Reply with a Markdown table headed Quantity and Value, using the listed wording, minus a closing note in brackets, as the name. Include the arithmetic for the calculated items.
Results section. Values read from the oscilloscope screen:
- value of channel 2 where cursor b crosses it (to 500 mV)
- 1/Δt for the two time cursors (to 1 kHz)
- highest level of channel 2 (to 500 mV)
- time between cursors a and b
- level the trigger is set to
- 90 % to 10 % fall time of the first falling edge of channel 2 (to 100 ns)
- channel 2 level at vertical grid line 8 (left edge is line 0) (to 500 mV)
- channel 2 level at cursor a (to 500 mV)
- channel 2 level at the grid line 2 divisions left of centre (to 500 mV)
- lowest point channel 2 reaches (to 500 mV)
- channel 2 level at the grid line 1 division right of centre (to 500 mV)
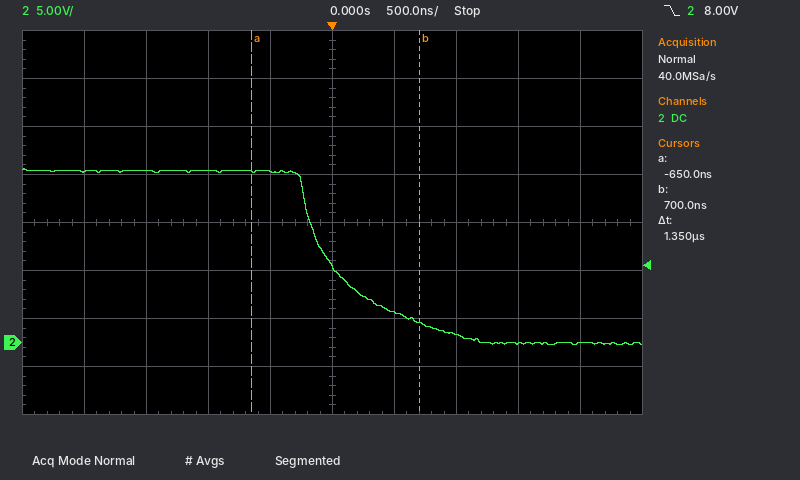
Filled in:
| Quantity | Value |
|---|---|
| value of channel 2 where cursor b crosses it | 2.0 V |
| 1/Δt for the two time cursors | 1 / 1.35 µs ≈ 741 kHz |
| highest level of channel 2 | 18.0 V |
| time between cursors a and b | 1.35 µs |
| level the trigger is set to | 8.00 V |
| 90 % to 10 % fall time of the first falling edge of channel 2 | 1.0 µs |
| channel 2 level at vertical grid line 8 (left edge is line 0) | 0.0 V |
| channel 2 level at cursor a | 18.0 V |
| channel 2 level at the grid line 2 divisions left of centre | 18.0 V |
| lowest point channel 2 reaches | 0.0 V |
| channel 2 level at the grid line 1 division right of centre | 3.0 V |
